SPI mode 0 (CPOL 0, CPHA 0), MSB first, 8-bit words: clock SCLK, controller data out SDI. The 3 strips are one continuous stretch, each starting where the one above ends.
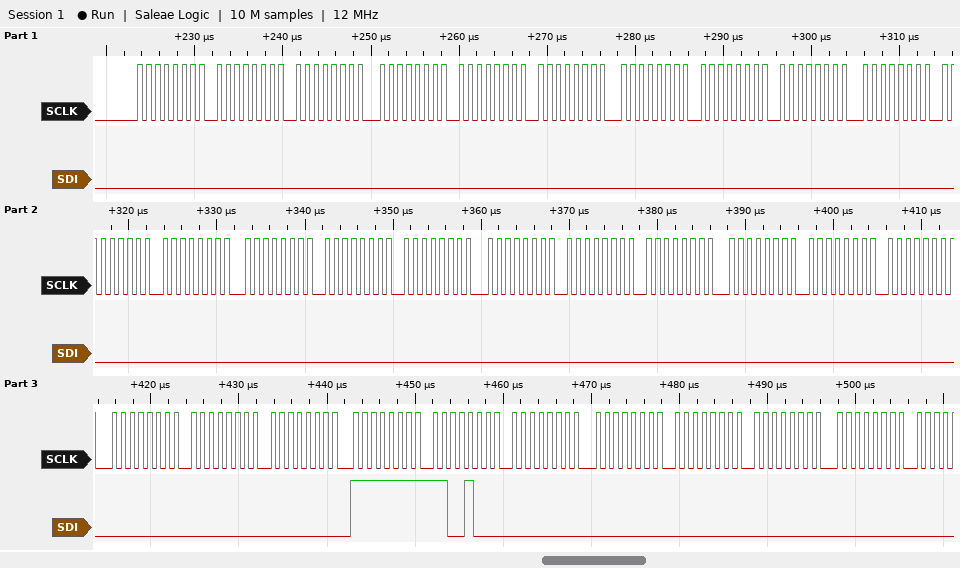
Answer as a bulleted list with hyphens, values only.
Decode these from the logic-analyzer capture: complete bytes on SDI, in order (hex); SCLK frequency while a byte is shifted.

- 00 00 00 00 00 00 00 00 00 00 00 00 00 00 00 00 00 00 00 00 00 00 00 00 FF C8 00 00 00 00 00
- 1 MHz
